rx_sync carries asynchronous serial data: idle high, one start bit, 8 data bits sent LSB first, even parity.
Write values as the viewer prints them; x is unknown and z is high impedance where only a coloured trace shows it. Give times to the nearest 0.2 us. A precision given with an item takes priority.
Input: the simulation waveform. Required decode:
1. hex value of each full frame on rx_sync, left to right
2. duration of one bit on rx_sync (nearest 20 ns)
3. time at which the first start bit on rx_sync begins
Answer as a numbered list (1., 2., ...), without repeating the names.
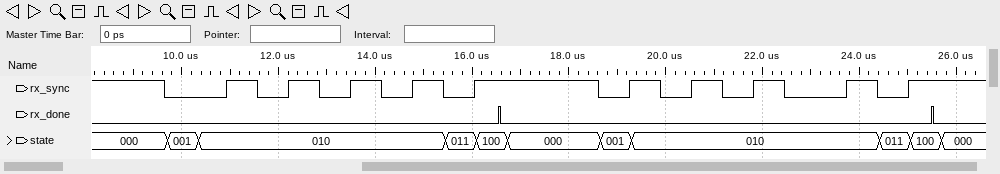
1. AA, 95
2. 640 ns
3. 9.6 us
